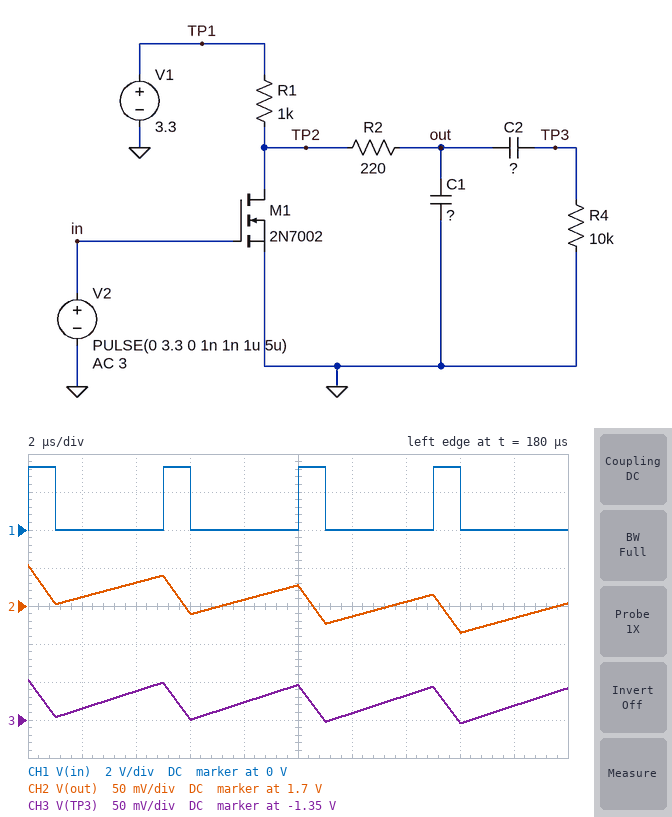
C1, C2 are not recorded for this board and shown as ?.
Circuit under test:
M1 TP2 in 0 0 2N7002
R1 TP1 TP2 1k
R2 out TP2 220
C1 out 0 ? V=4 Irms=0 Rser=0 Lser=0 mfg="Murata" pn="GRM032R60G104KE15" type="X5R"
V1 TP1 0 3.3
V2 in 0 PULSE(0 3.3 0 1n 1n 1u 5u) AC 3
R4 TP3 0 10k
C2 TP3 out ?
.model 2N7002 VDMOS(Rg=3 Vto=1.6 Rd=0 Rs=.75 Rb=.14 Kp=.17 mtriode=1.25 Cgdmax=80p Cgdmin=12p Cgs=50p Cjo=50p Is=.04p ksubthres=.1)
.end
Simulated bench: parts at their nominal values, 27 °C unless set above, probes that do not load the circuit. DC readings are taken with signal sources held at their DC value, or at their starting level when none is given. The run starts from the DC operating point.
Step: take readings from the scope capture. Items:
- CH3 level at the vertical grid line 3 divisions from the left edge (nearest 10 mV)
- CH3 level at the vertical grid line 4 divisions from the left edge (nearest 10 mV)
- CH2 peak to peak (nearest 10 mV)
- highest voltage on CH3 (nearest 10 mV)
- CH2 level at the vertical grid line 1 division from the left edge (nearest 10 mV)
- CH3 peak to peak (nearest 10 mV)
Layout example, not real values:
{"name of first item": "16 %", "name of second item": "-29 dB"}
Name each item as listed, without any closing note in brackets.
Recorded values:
{"CH3 level at the vertical grid line 3 divisions from the left edge": "-1.35 V", "CH3 level at the vertical grid line 4 divisions from the left edge": "-1.33 V", "CH2 peak to peak": "90 mV", "highest voltage on CH3": "-1.30 V", "CH2 level at the vertical grid line 1 division from the left edge": "1.71 V", "CH3 peak to peak": "60 mV"}
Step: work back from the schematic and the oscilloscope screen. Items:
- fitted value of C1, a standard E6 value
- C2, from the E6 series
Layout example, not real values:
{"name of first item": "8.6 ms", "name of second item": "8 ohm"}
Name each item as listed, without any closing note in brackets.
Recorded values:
{"fitted value of C1, a standard E6 value": "150 nF", "C2, from the E6 series": "68 nF"}
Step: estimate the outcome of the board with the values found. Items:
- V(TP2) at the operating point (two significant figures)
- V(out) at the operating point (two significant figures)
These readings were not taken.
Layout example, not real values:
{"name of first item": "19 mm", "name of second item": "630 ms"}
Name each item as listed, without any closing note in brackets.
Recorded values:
{"V(TP2) at the operating point": "3.3 V", "V(out) at the operating point": "3.3 V"}
